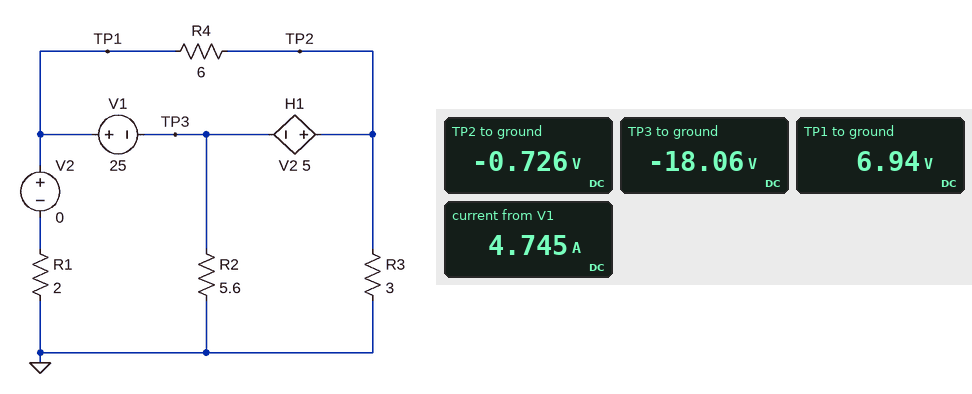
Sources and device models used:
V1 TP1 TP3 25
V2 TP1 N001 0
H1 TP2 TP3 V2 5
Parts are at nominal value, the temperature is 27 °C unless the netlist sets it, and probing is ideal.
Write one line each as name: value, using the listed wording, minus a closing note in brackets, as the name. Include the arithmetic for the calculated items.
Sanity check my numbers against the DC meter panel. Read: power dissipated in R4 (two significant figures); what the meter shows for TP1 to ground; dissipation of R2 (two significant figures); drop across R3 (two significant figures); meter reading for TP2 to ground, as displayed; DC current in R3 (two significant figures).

power dissipated in R4: (6.94 V - (-726 mV))^2 / 6 Ω = 9.8 W
what the meter shows for TP1 to ground: 6.94 V
dissipation of R2: (0 V - (-18.06 V))^2 / 5.6 Ω = 58 W
drop across R3: 0 V - (-726 mV) = 730 mV
meter reading for TP2 to ground, as displayed: -0.726 V
DC current in R3: (0 V - (-726 mV)) / 3 Ω = 240 mA
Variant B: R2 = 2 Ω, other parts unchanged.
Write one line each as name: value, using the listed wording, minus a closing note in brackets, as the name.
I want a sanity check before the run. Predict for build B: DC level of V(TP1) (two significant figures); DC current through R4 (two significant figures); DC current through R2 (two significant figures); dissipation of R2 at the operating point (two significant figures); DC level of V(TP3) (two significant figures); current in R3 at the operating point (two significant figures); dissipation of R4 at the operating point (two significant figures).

DC level of V(TP1): 9.6 V
DC current through R4: 160 mA
DC current through R2: 7.7 A
dissipation of R2 at the operating point: 120 W
DC level of V(TP3): -15 V
current in R3 at the operating point: 2.9 A
dissipation of R4 at the operating point: 150 mW
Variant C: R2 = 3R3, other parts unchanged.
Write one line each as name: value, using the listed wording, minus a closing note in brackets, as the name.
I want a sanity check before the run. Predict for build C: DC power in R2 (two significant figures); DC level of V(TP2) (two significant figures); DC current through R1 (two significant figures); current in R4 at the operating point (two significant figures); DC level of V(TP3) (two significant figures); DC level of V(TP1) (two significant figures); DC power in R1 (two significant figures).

DC power in R2: 87 W
DC level of V(TP2): 3.3 V
DC current through R1: 4.0 A
current in R4 at the operating point: 800 mA
DC level of V(TP3): -17 V
DC level of V(TP1): 8.1 V
DC power in R1: 33 W
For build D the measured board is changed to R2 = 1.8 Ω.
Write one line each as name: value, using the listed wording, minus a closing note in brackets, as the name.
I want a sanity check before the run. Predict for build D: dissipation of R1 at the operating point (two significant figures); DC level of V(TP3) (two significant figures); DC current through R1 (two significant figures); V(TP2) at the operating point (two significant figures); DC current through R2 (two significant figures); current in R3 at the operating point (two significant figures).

dissipation of R1 at the operating point: 50 W
DC level of V(TP3): -15 V
DC current through R1: 5.0 A
V(TP2) at the operating point: 10 V
DC current through R2: 8.3 A
current in R3 at the operating point: 3.3 A
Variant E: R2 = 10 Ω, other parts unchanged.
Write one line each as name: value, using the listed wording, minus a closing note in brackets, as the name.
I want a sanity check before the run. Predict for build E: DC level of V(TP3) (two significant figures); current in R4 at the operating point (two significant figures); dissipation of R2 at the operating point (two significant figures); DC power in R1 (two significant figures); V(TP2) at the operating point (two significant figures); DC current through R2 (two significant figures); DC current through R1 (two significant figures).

DC level of V(TP3): -19 V
current in R4 at the operating point: 1.6 A
dissipation of R2 at the operating point: 36 W
DC power in R1: 19 W
V(TP2) at the operating point: -3.5 V
DC current through R2: 1.9 A
DC current through R1: 3.1 A
